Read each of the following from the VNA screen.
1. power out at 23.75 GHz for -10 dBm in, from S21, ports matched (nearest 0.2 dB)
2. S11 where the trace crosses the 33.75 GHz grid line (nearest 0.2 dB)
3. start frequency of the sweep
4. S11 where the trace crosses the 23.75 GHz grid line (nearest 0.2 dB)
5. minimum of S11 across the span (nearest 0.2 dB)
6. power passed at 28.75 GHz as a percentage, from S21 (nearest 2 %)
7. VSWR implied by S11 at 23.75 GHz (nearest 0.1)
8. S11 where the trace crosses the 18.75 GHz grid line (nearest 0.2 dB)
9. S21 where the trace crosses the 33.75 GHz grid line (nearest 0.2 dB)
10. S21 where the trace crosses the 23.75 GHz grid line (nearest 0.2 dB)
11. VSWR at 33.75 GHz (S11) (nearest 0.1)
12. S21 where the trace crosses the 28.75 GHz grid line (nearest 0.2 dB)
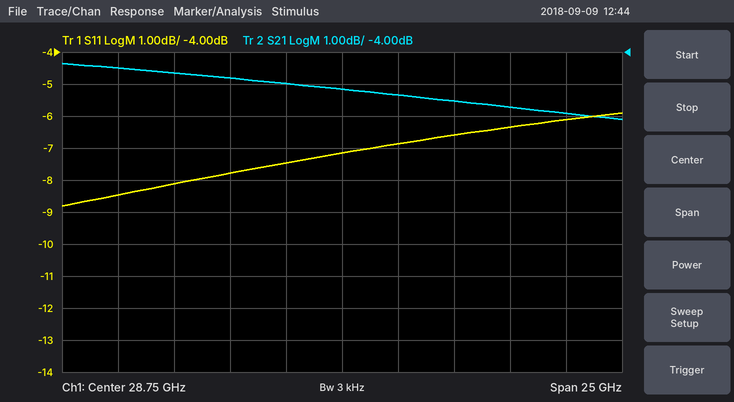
-14.8 dBm
-6.6 dB
16.25 GHz
-7.8 dB
-8.8 dB
30 %
2.4
-8.4 dB
-5.6 dB
-4.8 dB
2.8
-5.2 dB
